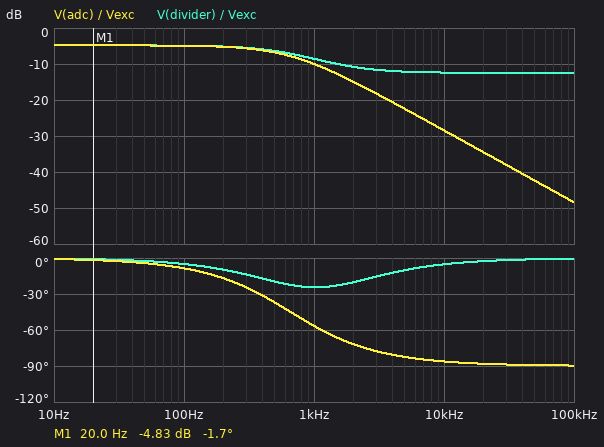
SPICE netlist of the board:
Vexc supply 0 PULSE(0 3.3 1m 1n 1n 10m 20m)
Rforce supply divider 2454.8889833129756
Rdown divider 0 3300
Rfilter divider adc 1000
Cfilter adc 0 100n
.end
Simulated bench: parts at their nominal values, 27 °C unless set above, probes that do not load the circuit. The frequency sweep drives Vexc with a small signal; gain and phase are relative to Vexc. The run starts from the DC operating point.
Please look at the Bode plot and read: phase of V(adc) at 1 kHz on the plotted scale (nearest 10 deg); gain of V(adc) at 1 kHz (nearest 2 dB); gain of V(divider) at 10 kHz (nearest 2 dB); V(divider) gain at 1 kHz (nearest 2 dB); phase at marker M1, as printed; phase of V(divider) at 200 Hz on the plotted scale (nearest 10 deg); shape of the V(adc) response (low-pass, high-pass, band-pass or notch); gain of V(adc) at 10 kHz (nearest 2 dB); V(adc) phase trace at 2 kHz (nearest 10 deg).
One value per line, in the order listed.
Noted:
-60 deg
-10 dB
-12 dB
-8 dB
-1.7 deg
-10 deg
low-pass
-28 dB
-70 deg
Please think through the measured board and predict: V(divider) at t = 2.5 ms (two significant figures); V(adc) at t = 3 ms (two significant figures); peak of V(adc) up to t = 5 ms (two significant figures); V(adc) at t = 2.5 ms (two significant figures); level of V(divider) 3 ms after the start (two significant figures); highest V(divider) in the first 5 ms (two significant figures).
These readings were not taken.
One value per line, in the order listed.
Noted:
1.9 V
1.9 V
1.9 V
1.9 V
1.9 V
1.9 V
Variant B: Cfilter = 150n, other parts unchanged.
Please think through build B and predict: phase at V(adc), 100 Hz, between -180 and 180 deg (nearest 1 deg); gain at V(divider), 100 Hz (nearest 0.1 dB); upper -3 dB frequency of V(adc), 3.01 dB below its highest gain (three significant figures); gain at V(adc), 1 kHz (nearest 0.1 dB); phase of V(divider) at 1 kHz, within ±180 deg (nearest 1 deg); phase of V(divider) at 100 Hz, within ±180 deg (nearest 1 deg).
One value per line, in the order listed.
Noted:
-13 deg
-5.0 dB
441 Hz
-12.7 dB
-23 deg
-7 deg
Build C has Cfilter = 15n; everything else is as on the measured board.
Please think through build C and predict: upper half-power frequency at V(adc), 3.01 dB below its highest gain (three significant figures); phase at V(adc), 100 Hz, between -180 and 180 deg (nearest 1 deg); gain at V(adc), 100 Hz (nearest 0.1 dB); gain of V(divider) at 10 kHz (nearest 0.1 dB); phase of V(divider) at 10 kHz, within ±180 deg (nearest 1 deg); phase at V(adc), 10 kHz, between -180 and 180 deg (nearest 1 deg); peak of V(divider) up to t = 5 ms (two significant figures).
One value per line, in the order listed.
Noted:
4.41 kHz
-1 deg
-4.8 dB
-10.0 dB
-23 deg
-66 deg
1.9 V
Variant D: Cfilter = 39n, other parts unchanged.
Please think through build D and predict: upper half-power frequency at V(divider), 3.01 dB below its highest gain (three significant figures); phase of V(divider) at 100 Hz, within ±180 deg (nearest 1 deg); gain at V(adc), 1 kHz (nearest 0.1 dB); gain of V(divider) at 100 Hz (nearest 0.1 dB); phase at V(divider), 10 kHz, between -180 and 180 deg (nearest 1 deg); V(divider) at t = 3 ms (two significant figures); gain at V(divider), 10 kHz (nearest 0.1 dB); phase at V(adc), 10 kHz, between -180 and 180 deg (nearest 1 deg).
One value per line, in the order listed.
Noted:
2.09 kHz
-2 deg
-6.1 dB
-4.8 dB
-13 deg
1.9 V
-11.9 dB
-80 deg
